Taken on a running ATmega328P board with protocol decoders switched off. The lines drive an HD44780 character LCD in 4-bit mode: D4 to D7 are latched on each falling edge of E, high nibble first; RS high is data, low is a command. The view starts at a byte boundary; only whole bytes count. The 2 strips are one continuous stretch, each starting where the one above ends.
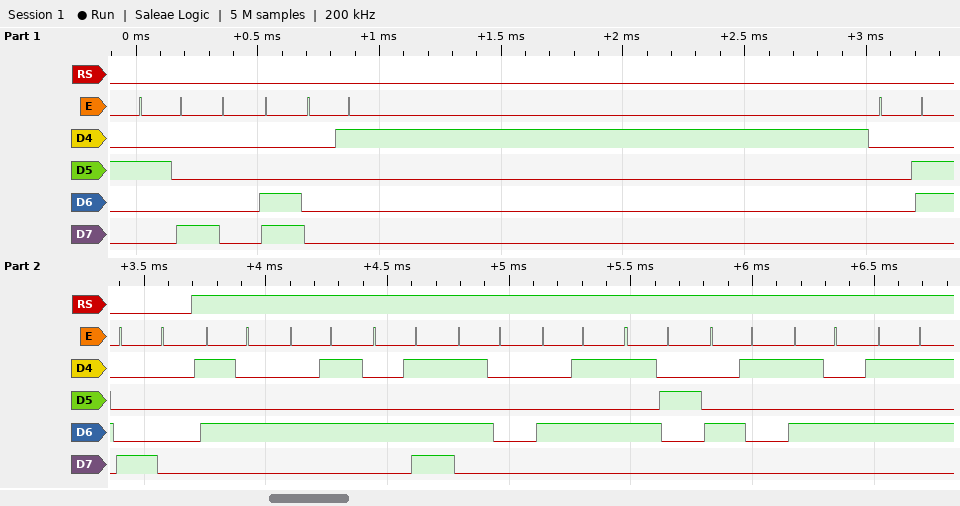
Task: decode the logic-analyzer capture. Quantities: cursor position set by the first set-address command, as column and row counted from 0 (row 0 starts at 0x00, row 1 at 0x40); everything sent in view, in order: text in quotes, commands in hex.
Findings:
column 0, row 0
0x28 0x0C 0x01 0x06 0x80 "TEMPERATU"
